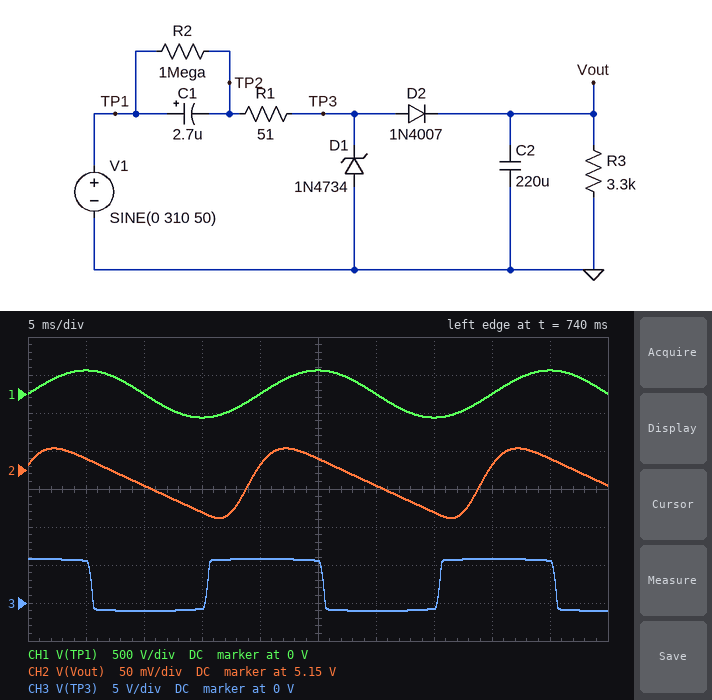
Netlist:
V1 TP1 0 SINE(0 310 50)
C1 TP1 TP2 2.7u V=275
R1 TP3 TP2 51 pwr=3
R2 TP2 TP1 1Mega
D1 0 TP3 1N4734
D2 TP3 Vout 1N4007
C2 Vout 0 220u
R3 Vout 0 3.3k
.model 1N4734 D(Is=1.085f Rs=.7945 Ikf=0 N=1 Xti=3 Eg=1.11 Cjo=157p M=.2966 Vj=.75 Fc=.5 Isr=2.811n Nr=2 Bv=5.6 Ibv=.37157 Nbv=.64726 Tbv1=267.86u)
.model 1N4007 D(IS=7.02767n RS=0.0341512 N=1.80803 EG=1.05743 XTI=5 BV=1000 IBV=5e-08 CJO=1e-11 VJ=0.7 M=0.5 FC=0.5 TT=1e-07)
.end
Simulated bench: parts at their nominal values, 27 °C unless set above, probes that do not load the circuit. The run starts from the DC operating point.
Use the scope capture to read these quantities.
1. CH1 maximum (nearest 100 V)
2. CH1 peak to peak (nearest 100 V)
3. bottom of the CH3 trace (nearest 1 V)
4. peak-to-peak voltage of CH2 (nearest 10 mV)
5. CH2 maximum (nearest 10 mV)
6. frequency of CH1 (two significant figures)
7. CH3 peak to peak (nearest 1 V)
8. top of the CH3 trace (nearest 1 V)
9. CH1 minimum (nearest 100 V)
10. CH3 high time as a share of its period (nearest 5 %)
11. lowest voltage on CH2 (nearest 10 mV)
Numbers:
300 V
600 V
-1 V
90 mV
5.18 V
50 Hz
7 V
6 V
-300 V
50 %
5.09 V
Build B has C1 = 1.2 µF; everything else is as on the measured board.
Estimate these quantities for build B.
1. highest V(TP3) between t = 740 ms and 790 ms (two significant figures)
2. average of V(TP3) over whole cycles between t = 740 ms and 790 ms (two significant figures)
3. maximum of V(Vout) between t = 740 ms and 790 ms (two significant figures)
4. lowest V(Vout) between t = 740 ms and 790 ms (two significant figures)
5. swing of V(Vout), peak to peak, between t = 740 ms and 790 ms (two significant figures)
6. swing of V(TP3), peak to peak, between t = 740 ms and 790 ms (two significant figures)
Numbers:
5.7 V
2.4 V
5.1 V
5.0 V
82 mV
6.6 V
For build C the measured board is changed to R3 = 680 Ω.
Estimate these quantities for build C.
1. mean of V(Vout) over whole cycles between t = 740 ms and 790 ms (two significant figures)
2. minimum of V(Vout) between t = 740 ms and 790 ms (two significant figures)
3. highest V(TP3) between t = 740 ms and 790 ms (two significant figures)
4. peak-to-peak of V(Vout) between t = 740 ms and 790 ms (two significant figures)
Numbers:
5.0 V
4.7 V
5.8 V
420 mV
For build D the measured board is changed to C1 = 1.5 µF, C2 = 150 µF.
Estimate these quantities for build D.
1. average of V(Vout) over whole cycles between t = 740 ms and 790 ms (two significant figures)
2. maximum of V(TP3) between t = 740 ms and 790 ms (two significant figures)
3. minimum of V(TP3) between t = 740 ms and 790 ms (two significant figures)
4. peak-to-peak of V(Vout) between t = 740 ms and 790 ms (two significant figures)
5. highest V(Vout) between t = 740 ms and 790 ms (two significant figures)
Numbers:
5.0 V
5.7 V
-950 mV
120 mV
5.1 V
